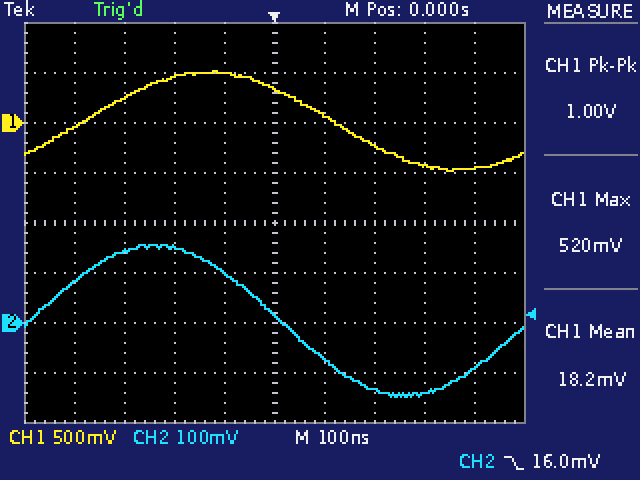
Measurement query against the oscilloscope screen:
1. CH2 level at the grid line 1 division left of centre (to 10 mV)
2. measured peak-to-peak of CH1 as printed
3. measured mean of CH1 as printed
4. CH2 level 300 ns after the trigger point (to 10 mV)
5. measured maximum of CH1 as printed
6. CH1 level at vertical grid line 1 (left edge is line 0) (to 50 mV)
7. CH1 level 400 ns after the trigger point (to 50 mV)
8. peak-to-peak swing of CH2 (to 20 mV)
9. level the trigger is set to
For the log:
100 mV
1.00 V
18.2 mV
-140 mV
520 mV
-50 mV
-450 mV
300 mV
16.0 mV
